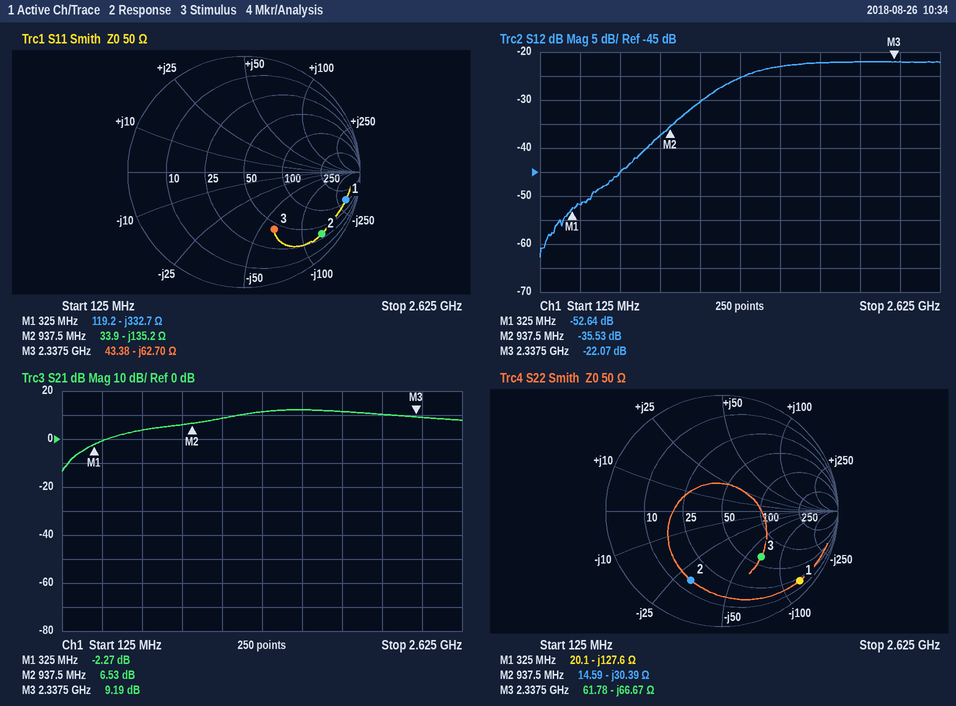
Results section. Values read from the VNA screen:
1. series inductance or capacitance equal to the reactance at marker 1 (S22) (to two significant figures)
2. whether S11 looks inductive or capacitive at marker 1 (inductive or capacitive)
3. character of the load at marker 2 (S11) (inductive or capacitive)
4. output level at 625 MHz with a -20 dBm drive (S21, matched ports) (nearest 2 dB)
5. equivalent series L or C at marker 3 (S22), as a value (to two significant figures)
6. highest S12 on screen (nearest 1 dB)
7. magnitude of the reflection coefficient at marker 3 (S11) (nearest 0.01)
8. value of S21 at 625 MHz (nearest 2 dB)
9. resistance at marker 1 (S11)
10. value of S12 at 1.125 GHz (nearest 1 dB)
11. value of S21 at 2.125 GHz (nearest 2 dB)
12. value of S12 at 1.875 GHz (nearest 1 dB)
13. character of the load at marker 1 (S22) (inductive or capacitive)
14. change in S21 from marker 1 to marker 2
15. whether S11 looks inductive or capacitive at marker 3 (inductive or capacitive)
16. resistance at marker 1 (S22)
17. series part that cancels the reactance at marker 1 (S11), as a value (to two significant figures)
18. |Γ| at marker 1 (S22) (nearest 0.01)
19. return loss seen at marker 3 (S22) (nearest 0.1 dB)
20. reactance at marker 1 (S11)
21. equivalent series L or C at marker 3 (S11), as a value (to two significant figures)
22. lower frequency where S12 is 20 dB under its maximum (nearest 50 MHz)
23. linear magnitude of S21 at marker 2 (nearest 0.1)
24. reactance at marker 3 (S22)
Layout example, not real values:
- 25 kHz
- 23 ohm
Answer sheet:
- 3.8 pF
- capacitive
- capacitive
- -16 dBm
- 1.0 pF
- -22 dB
- 0.56
- 4 dB
- 119.2 Ω
- -30 dB
- 10 dB
- -22 dB
- capacitive
- 8.80 dB
- capacitive
- 20.1 Ω
- 160 nH
- 0.90
- 5.7 dB
- -332.7 Ω
- 1.1 pF
- 750 MHz
- 2.1
- -66.67 Ω
